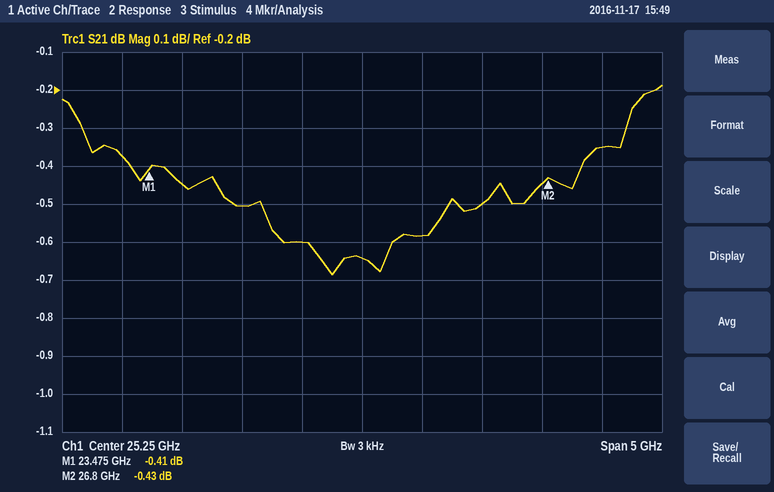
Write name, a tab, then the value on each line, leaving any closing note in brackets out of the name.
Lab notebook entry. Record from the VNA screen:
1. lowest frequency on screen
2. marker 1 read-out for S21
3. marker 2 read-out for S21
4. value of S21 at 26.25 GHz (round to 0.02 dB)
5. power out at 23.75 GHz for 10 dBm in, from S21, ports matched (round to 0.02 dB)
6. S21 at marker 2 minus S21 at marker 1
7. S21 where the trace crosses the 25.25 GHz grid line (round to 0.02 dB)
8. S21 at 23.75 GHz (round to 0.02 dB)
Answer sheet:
lowest frequency on screen	22.75 GHz
marker 1 read-out for S21	-0.41 dB
marker 2 read-out for S21	-0.43 dB
value of S21 at 26.25 GHz	-0.50 dB
power out at 23.75 GHz for 10 dBm in, from S21, ports matched	9.56 dBm
S21 at marker 2 minus S21 at marker 1	-0.02 dB
S21 where the trace crosses the 25.25 GHz grid line	-0.64 dB
S21 at 23.75 GHz	-0.44 dB
